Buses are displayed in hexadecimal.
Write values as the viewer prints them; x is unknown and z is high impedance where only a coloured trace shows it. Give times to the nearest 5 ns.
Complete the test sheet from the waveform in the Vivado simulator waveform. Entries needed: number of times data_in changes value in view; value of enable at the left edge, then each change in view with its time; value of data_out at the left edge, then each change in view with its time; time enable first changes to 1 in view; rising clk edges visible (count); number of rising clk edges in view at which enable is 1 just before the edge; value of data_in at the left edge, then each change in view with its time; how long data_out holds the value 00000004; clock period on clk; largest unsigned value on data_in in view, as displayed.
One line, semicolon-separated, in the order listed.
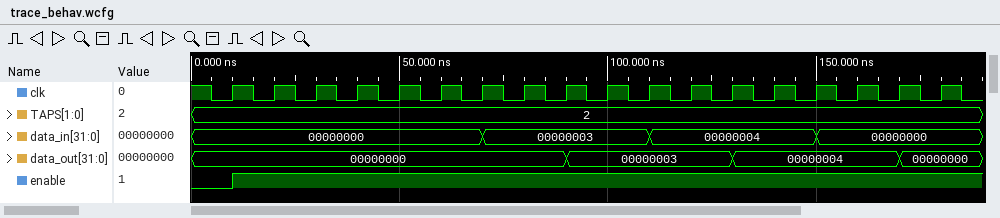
3; 0, 1 at 10 ns; 00000000, 00000003 at 90 ns, 00000004 at 130 ns, 00000000 at 170 ns; 10 ns; 18; 17; 00000000, 00000003 at 70 ns, 00000004 at 110 ns, 00000000 at 150 ns; 40 ns; 10 ns; 00000004
